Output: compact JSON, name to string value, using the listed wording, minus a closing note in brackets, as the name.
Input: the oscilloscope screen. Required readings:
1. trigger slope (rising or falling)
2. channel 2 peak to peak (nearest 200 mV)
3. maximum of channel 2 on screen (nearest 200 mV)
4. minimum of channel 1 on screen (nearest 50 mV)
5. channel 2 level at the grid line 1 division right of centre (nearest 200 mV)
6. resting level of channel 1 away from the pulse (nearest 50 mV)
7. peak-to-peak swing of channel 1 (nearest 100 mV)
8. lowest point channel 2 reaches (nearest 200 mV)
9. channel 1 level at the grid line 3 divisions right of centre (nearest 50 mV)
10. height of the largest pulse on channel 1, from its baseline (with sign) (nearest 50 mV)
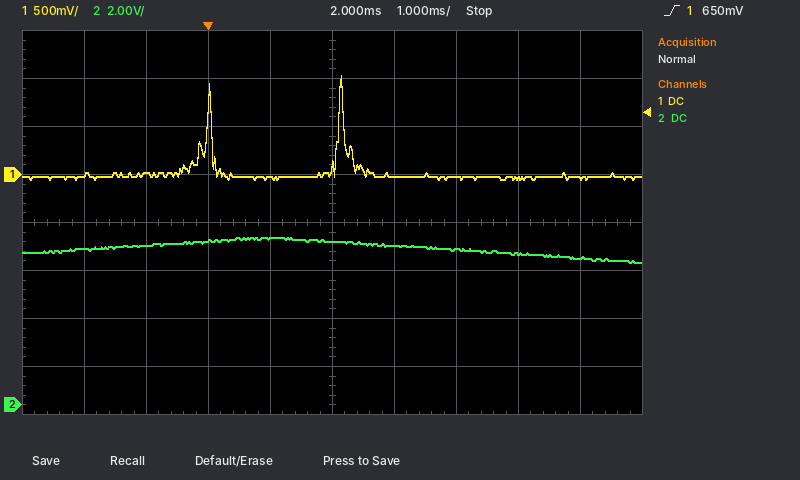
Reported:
{"trigger slope": "rising", "channel 2 peak to peak": "1.0 V", "maximum of channel 2 on screen": "7.0 V", "minimum of channel 1 on screen": "-50 mV", "channel 2 level at the grid line 1 division right of centre": "6.6 V", "resting level of channel 1 away from the pulse": "0 mV", "peak-to-peak swing of channel 1": "1.10 V", "lowest point channel 2 reaches": "6.0 V", "channel 1 level at the grid line 3 divisions right of centre": "-50 mV", "height of the largest pulse on channel 1, from its baseline (with sign)": "+1.05 V"}
